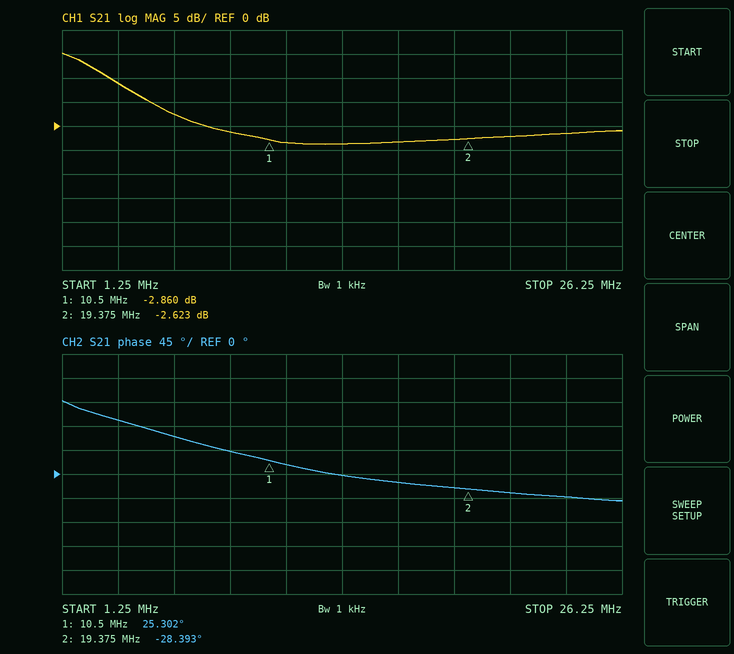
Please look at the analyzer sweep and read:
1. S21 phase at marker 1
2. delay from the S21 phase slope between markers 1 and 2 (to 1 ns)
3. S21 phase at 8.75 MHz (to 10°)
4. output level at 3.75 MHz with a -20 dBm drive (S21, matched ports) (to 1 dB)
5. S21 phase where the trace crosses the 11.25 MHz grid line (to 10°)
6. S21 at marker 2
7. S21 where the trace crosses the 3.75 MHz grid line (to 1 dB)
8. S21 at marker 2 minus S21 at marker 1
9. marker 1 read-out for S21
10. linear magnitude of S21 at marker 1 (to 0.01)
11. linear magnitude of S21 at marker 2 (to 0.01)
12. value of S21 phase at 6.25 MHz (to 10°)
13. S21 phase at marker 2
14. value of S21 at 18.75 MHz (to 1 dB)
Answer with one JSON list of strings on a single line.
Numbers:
["25.302°", "17 ns", "40°", "-11 dBm", "20°", "-2.623 dB", "9 dB", "0.237 dB", "-2.860 dB", "0.72", "0.74", "70°", "-28.393°", "-3 dB"]
